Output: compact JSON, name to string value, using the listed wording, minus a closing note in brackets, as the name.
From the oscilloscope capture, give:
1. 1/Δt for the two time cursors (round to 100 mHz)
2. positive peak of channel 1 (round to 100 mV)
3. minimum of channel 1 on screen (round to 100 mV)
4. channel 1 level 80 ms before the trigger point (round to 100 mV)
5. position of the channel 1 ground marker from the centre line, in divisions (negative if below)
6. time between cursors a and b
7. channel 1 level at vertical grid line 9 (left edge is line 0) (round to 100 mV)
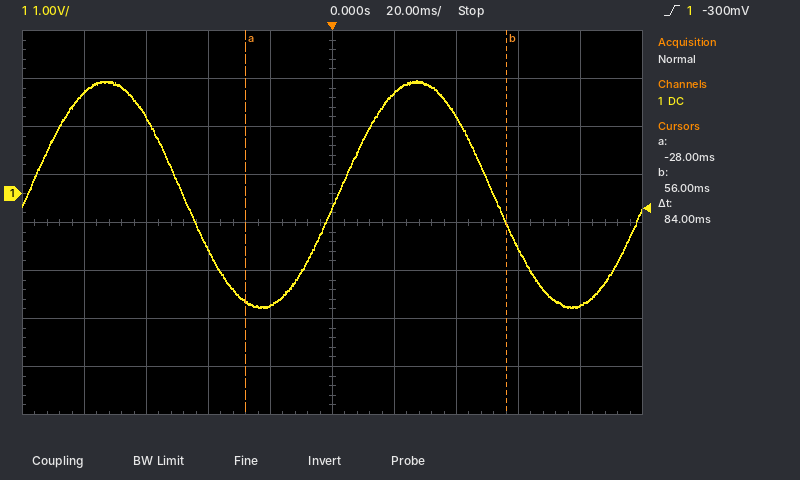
{"1/Δt for the two time cursors": "11.9 Hz", "positive peak of channel 1": "2.4 V", "minimum of channel 1 on screen": "-2.4 V", "channel 1 level 80 ms before the trigger point": "2.1 V", "position of the channel 1 ground marker from the centre line, in divisions": "+0.6 div", "time between cursors a and b": "84 ms", "channel 1 level at vertical grid line 9 (left edge is line 0)": "-2.3 V"}
